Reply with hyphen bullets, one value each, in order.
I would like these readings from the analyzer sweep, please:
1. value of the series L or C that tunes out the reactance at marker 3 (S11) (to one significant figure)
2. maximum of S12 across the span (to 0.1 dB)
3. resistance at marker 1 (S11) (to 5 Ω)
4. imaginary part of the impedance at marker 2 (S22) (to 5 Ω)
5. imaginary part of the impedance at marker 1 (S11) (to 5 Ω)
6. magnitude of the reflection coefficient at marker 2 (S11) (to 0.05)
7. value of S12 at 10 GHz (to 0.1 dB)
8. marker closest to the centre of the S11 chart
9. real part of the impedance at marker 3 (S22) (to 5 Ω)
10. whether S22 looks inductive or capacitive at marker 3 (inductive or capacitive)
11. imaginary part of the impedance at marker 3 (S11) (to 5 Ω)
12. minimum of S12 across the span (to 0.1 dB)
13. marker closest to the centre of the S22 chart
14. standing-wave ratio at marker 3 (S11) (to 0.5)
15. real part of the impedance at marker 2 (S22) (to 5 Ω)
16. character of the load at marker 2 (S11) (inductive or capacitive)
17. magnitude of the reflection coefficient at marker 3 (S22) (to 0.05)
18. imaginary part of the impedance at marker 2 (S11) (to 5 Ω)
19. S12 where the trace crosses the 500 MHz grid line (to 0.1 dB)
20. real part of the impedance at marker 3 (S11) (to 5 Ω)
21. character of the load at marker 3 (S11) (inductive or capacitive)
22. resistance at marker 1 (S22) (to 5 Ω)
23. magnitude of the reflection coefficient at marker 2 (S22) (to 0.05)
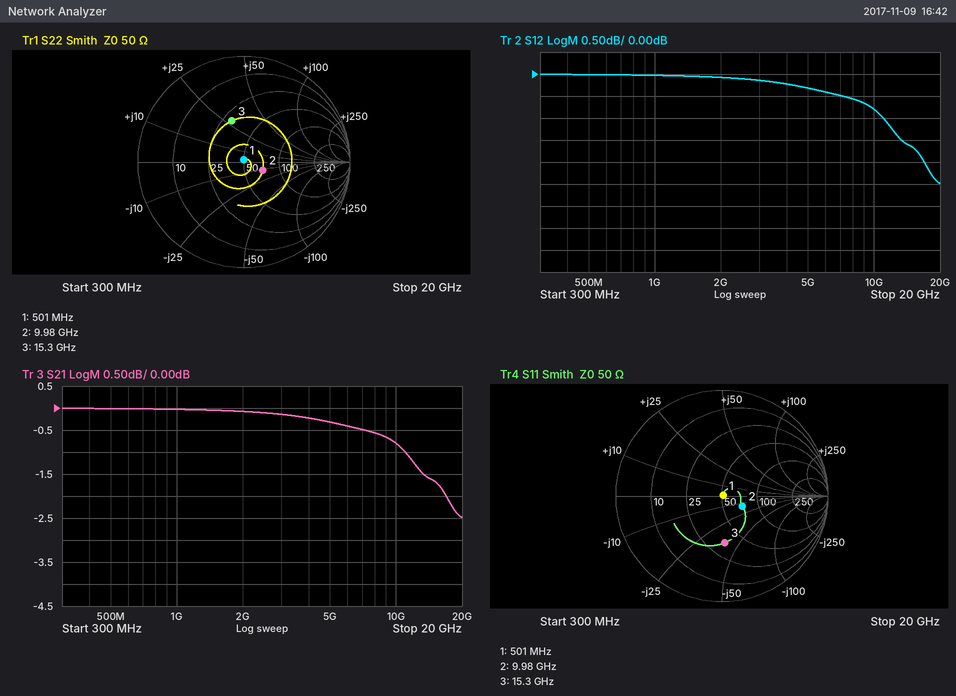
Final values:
- 400 pH
- 0.0 dB
- 50 Ω
- -10 Ω
- 0 Ω
- 0.20
- -0.8 dB
- marker 1
- 30 Ω
- inductive
- -40 Ω
- -2.5 dB
- marker 1
- 2.5
- 70 Ω
- capacitive
- 0.40
- -15 Ω
- 0.0 dB
- 35 Ω
- capacitive
- 50 Ω
- 0.20
